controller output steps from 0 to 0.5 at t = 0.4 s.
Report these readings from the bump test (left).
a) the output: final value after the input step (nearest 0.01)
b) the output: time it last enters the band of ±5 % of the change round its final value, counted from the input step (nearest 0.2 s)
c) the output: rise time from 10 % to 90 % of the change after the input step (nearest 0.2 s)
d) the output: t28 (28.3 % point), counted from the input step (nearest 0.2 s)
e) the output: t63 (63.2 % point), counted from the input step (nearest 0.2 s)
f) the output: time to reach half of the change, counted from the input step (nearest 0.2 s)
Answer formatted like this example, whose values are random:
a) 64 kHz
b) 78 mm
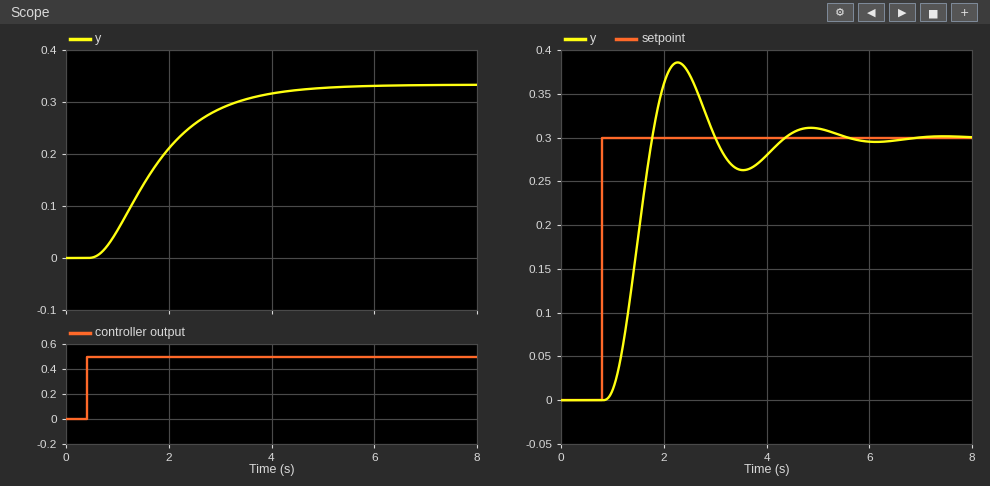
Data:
a) 0.33
b) 3.6 s
c) 2.4 s
d) 0.8 s
e) 1.6 s
f) 1.2 s
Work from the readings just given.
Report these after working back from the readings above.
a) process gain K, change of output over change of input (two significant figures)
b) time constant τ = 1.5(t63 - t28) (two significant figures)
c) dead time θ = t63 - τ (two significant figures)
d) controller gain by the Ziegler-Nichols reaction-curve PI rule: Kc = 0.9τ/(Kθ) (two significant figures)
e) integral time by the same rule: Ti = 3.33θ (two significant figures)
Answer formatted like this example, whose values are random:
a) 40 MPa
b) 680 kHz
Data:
a) 0.66
b) 1.2 s
c) 0.40 s
d) 4.1
e) 1.3 s
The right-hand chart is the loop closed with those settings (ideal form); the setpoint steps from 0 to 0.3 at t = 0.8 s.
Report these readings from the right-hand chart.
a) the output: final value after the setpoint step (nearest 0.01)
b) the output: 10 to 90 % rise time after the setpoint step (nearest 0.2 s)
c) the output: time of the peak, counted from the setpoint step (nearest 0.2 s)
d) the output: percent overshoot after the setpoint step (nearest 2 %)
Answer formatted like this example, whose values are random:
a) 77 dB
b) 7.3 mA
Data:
a) 0.30
b) 0.6 s
c) 1.4 s
d) 28 %
